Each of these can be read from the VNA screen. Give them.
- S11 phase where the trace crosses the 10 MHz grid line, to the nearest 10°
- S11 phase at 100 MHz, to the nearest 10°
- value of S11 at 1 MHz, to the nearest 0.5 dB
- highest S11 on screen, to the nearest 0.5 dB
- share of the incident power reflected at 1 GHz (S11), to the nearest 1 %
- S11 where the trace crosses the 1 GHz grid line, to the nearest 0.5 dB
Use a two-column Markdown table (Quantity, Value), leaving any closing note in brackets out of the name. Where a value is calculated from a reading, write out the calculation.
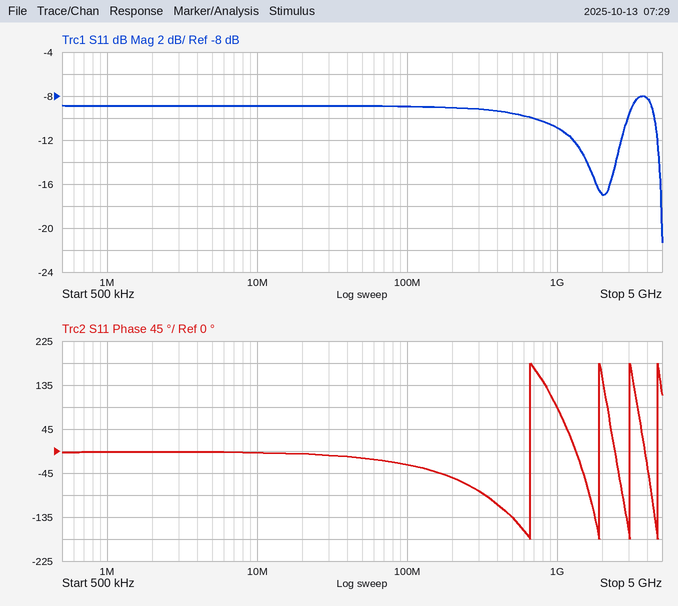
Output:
| Quantity | Value |
|---|---|
| S11 phase where the trace crosses the 10 MHz grid line, to the nearest 10° | 0° |
| S11 phase at 100 MHz, to the nearest 10° | -30° |
| value of S11 at 1 MHz, to the nearest 0.5 dB | -9.0 dB |
| highest S11 on screen, to the nearest 0.5 dB | -8.0 dB |
| share of the incident power reflected at 1 GHz (S11), to the nearest 1 % | 10^(-11/10) ≈ 8 % |
| S11 where the trace crosses the 1 GHz grid line, to the nearest 0.5 dB | -11.0 dB |
